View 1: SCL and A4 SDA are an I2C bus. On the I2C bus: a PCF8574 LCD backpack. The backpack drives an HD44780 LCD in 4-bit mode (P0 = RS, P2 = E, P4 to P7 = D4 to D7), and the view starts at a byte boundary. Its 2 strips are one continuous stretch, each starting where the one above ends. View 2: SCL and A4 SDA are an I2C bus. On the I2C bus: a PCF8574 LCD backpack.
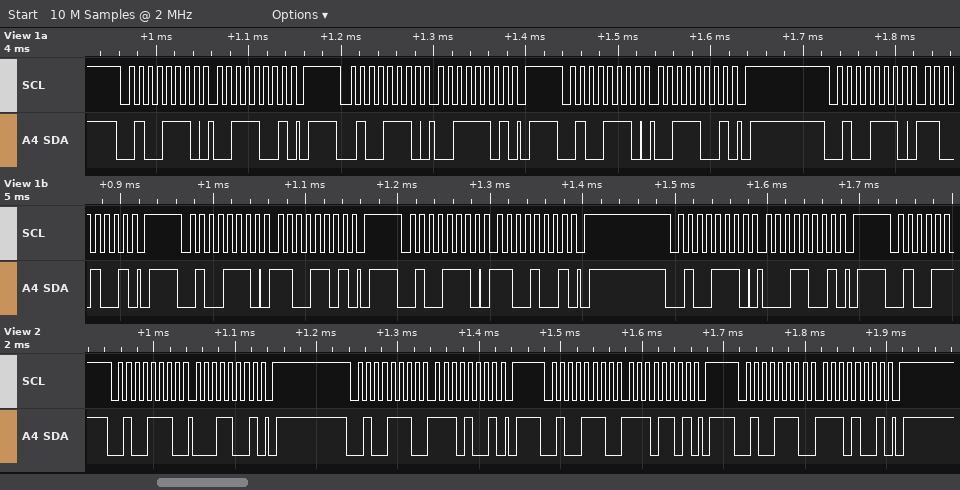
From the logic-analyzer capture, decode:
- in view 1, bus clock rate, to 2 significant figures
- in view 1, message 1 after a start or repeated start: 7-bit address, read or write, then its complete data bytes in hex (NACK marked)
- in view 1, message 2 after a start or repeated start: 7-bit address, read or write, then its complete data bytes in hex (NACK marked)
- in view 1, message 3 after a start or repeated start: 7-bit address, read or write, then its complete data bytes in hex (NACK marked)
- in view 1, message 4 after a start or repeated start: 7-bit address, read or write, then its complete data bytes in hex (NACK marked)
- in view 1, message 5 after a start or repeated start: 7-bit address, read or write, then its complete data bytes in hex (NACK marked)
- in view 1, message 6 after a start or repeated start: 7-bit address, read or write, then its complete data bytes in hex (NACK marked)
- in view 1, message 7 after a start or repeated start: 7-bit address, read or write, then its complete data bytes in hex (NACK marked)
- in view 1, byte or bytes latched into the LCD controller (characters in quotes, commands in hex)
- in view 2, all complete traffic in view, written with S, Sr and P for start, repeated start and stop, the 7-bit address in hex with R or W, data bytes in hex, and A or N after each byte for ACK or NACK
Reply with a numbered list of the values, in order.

1. 100 kHz
2. 0x27 write: 39
3. 0x27 write: 3D
4. 0x27 write: 39
5. 0x27 write: C9
6. 0x27 write: CD
7. 0x27 write: C9
8. 0x27 write: 19
9. '<'
10. S 27W A 19 A P S 27W A E9 A P S 27W A ED A P S 27W A E9 A P
